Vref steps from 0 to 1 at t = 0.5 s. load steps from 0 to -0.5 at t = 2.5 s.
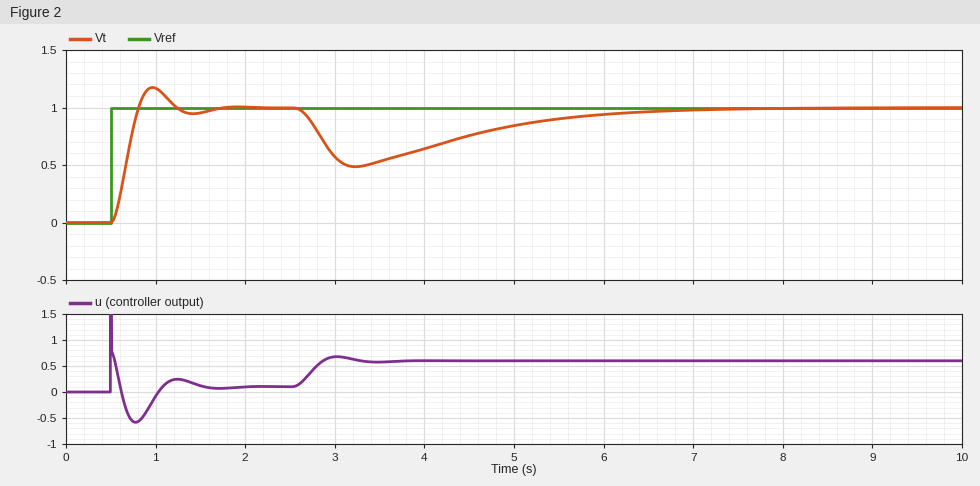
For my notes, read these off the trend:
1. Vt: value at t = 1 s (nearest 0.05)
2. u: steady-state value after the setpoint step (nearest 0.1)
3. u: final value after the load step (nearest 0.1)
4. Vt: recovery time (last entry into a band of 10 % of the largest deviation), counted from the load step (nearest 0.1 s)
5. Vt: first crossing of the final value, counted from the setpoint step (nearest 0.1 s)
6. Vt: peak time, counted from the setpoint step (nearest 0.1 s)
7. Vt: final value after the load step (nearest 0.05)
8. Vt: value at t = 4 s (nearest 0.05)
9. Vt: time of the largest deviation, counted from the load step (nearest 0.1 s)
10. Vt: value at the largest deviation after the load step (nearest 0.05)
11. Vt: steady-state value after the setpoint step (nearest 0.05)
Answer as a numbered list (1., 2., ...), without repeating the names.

1. 1.15
2. 0.1
3. 0.6
4. 3.7 s
5. 0.3 s
6. 0.5 s
7. 1.00
8. 0.65
9. 0.7 s
10. 0.50
11. 1.00
